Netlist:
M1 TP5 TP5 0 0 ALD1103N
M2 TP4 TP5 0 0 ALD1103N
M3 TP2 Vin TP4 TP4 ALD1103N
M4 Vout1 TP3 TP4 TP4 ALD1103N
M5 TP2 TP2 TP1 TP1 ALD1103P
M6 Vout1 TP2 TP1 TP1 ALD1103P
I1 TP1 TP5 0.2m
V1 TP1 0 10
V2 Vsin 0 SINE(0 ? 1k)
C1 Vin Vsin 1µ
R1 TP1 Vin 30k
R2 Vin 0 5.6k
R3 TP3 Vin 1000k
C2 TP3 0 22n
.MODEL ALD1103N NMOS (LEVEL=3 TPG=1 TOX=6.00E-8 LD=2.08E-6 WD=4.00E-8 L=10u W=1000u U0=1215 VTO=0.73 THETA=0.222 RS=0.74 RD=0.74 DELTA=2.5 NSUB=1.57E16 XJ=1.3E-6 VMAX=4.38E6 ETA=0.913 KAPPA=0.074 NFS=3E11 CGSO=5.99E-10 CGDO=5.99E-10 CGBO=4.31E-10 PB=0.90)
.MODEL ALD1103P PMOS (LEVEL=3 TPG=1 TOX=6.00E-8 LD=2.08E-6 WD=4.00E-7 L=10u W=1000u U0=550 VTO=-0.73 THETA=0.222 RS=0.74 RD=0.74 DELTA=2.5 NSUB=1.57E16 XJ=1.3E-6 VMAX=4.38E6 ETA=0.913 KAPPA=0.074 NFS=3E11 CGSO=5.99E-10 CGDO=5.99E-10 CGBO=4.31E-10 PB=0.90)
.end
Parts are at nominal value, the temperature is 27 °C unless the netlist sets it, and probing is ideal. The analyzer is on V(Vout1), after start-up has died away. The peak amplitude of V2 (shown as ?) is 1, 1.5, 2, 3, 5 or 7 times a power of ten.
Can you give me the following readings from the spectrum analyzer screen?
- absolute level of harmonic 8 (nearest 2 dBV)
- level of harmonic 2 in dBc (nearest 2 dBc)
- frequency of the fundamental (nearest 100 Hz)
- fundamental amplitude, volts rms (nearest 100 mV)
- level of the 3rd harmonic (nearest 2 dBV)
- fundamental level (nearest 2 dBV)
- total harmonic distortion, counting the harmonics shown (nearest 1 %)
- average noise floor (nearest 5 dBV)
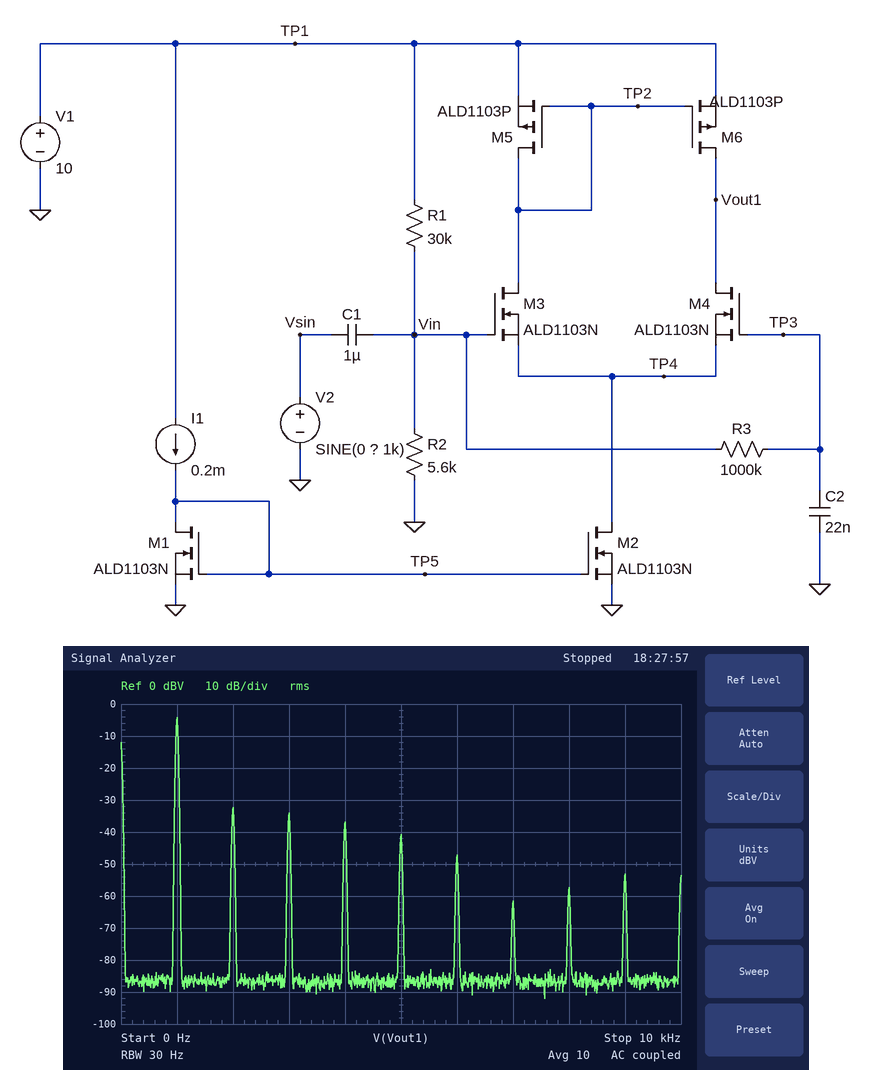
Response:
-58 dBV
-28 dBc
1.0 kHz
600 mV
-34 dBV
-4 dBV
6 %
-85 dBV
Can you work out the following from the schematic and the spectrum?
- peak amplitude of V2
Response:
10 mV
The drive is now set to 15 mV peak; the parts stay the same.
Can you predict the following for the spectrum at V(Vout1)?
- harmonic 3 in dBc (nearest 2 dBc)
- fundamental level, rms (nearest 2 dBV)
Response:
-22 dBc
-2 dBV
